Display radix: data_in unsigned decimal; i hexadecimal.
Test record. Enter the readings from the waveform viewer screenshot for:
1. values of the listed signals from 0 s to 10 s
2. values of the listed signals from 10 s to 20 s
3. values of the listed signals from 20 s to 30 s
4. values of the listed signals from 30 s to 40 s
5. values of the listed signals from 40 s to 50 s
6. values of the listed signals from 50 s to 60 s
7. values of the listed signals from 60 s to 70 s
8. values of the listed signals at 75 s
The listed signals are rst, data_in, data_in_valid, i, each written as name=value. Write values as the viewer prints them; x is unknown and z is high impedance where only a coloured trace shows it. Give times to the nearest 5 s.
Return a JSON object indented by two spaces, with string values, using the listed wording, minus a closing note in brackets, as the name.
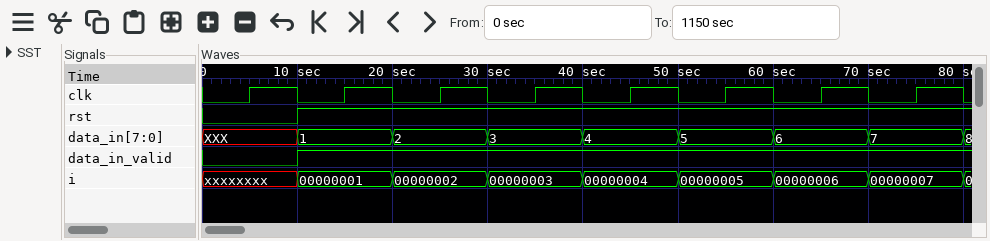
{
  "values of the listed signals from 0 s to 10 s": "rst=0, data_in=XXX, data_in_valid=0, i=xxxxxxxx",
  "values of the listed signals from 10 s to 20 s": "rst=1, data_in=1, data_in_valid=1, i=00000001",
  "values of the listed signals from 20 s to 30 s": "rst=1, data_in=2, data_in_valid=1, i=00000002",
  "values of the listed signals from 30 s to 40 s": "rst=1, data_in=3, data_in_valid=1, i=00000003",
  "values of the listed signals from 40 s to 50 s": "rst=1, data_in=4, data_in_valid=1, i=00000004",
  "values of the listed signals from 50 s to 60 s": "rst=1, data_in=5, data_in_valid=1, i=00000005",
  "values of the listed signals from 60 s to 70 s": "rst=1, data_in=6, data_in_valid=1, i=00000006",
  "values of the listed signals at 75 s": "rst=1, data_in=7, data_in_valid=1, i=00000007"
}
